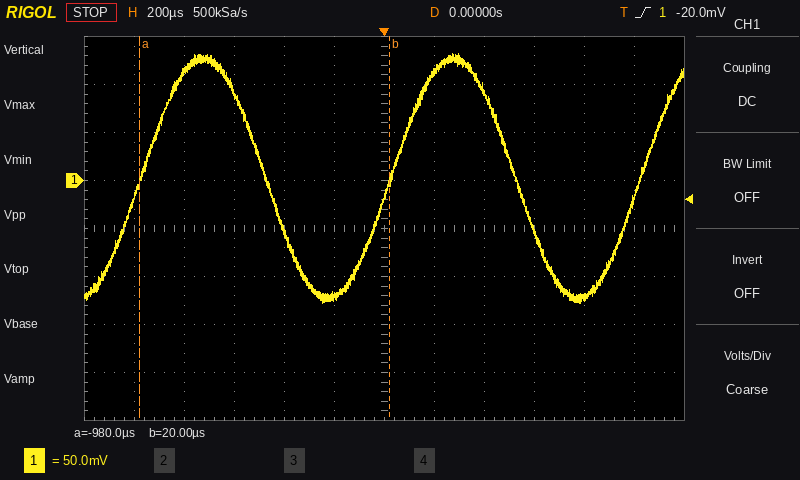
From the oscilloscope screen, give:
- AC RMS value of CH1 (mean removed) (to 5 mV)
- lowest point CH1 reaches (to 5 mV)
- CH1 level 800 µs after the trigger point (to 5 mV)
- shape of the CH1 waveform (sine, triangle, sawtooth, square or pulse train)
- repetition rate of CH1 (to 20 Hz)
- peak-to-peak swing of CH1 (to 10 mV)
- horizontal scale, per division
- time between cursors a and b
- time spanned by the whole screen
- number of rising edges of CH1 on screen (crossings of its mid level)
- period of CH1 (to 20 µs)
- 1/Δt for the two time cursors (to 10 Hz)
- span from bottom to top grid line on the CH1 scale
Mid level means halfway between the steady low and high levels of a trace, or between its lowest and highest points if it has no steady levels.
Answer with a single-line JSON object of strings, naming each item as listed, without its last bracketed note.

{"AC RMS value of CH1 (mean removed)": "90 mV", "lowest point CH1 reaches": "-130 mV", "CH1 level 800 µs after the trigger point": "-120 mV", "shape of the CH1 waveform": "sine", "repetition rate of CH1": "1.00 kHz", "peak-to-peak swing of CH1": "260 mV", "horizontal scale, per division": "200 µs", "time between cursors a and b": "1.00 ms", "time spanned by the whole screen": "2.4 ms", "number of rising edges of CH1 on screen": "3", "period of CH1": "1.00 ms", "1/Δt for the two time cursors": "1.00 kHz", "span from bottom to top grid line on the CH1 scale": "400 mV"}
